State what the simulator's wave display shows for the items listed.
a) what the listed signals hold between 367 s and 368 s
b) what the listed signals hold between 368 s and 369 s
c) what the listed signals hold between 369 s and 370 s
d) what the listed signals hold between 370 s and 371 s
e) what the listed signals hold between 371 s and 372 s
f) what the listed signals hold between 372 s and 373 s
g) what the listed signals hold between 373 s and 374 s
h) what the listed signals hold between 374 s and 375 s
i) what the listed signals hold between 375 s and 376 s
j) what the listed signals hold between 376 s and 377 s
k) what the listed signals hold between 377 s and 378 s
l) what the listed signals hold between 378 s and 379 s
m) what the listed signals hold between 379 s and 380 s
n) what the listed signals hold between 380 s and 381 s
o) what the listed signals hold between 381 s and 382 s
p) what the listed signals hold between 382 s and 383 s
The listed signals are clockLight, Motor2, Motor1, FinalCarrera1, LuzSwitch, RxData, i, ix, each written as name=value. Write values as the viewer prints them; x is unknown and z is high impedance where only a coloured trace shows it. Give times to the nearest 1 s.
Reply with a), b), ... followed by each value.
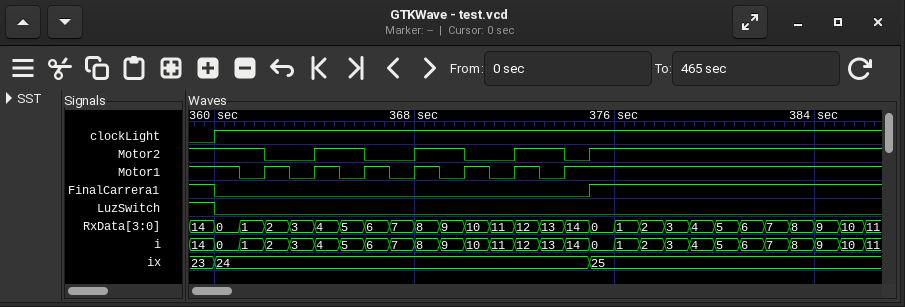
a) clockLight=1, Motor2=0, Motor1=0, FinalCarrera1=0, LuzSwitch=0, RxData=7, i=7, ix=24
b) clockLight=1, Motor2=1, Motor1=1, FinalCarrera1=0, LuzSwitch=0, RxData=8, i=8, ix=24
c) clockLight=1, Motor2=1, Motor1=0, FinalCarrera1=0, LuzSwitch=0, RxData=9, i=9, ix=24
d) clockLight=1, Motor2=0, Motor1=1, FinalCarrera1=0, LuzSwitch=0, RxData=10, i=10, ix=24
e) clockLight=1, Motor2=0, Motor1=0, FinalCarrera1=0, LuzSwitch=0, RxData=11, i=11, ix=24
f) clockLight=1, Motor2=1, Motor1=1, FinalCarrera1=0, LuzSwitch=0, RxData=12, i=12, ix=24
g) clockLight=1, Motor2=1, Motor1=0, FinalCarrera1=0, LuzSwitch=0, RxData=13, i=13, ix=24
h) clockLight=1, Motor2=0, Motor1=1, FinalCarrera1=0, LuzSwitch=0, RxData=14, i=14, ix=24
i) clockLight=1, Motor2=1, Motor1=1, FinalCarrera1=1, LuzSwitch=0, RxData=0, i=0, ix=25
j) clockLight=1, Motor2=1, Motor1=1, FinalCarrera1=1, LuzSwitch=0, RxData=1, i=1, ix=25
k) clockLight=1, Motor2=1, Motor1=1, FinalCarrera1=1, LuzSwitch=0, RxData=2, i=2, ix=25
l) clockLight=1, Motor2=1, Motor1=1, FinalCarrera1=1, LuzSwitch=0, RxData=3, i=3, ix=25
m) clockLight=1, Motor2=1, Motor1=1, FinalCarrera1=1, LuzSwitch=0, RxData=4, i=4, ix=25
n) clockLight=1, Motor2=1, Motor1=1, FinalCarrera1=1, LuzSwitch=0, RxData=5, i=5, ix=25
o) clockLight=1, Motor2=1, Motor1=1, FinalCarrera1=1, LuzSwitch=0, RxData=6, i=6, ix=25
p) clockLight=1, Motor2=1, Motor1=1, FinalCarrera1=1, LuzSwitch=0, RxData=7, i=7, ix=25
